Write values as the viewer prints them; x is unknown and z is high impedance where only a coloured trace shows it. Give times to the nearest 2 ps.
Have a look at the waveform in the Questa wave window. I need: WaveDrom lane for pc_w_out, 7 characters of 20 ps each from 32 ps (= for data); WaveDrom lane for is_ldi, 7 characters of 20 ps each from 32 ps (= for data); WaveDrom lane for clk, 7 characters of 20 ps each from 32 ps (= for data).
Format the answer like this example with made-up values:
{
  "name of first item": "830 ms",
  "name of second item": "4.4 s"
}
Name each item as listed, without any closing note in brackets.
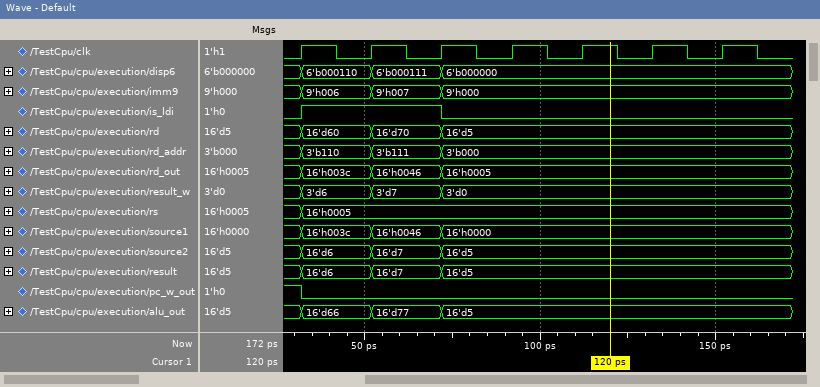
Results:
{
  "WaveDrom lane for pc_w_out, 7 characters of 20 ps each from 32 ps": "{name: 'pc_w_out', wave: '0......'}",
  "WaveDrom lane for is_ldi, 7 characters of 20 ps each from 32 ps": "{name: 'is_ldi', wave: '1.0....'}",
  "WaveDrom lane for clk, 7 characters of 20 ps each from 32 ps": "{name: 'clk', wave: 'p......'}"
}
